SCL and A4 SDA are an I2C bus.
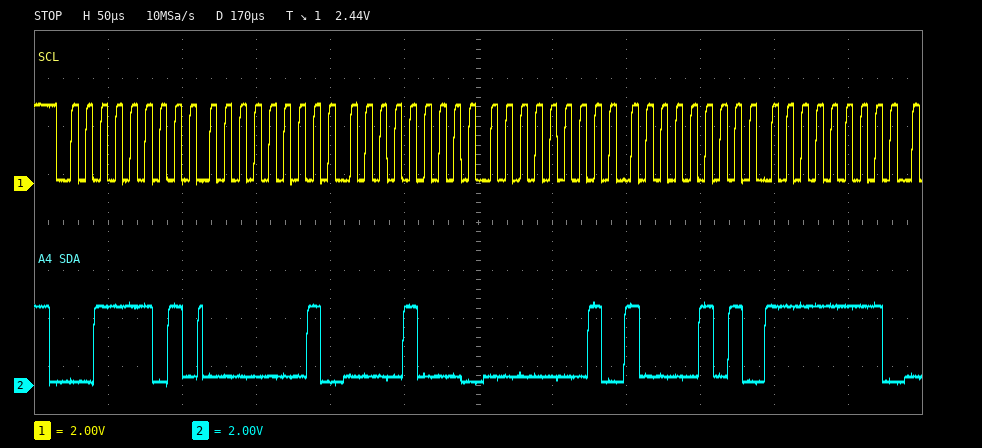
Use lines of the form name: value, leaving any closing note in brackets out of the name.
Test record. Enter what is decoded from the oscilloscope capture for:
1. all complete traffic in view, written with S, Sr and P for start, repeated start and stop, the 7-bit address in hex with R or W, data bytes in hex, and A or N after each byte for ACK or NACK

all complete traffic in view, written with S, Sr and P for start, repeated start and stop, the 7-bit address in hex with R or W, data bytes in hex, and A or N after each byte for ACK or NACK: S 1ER A 01 A 08 A 01 A 85 A FF A
